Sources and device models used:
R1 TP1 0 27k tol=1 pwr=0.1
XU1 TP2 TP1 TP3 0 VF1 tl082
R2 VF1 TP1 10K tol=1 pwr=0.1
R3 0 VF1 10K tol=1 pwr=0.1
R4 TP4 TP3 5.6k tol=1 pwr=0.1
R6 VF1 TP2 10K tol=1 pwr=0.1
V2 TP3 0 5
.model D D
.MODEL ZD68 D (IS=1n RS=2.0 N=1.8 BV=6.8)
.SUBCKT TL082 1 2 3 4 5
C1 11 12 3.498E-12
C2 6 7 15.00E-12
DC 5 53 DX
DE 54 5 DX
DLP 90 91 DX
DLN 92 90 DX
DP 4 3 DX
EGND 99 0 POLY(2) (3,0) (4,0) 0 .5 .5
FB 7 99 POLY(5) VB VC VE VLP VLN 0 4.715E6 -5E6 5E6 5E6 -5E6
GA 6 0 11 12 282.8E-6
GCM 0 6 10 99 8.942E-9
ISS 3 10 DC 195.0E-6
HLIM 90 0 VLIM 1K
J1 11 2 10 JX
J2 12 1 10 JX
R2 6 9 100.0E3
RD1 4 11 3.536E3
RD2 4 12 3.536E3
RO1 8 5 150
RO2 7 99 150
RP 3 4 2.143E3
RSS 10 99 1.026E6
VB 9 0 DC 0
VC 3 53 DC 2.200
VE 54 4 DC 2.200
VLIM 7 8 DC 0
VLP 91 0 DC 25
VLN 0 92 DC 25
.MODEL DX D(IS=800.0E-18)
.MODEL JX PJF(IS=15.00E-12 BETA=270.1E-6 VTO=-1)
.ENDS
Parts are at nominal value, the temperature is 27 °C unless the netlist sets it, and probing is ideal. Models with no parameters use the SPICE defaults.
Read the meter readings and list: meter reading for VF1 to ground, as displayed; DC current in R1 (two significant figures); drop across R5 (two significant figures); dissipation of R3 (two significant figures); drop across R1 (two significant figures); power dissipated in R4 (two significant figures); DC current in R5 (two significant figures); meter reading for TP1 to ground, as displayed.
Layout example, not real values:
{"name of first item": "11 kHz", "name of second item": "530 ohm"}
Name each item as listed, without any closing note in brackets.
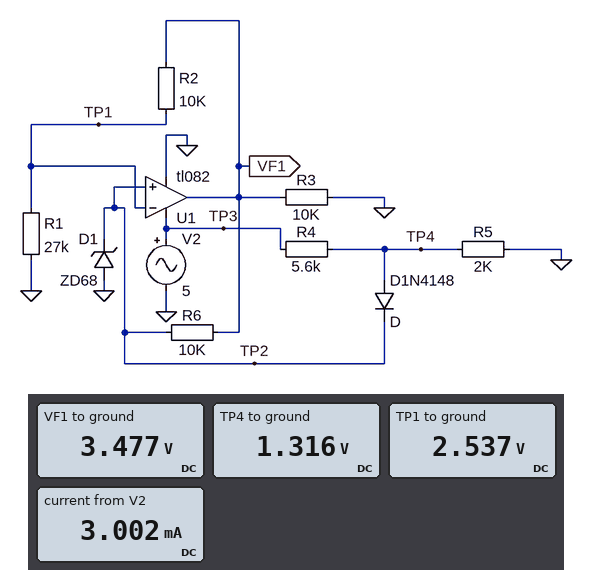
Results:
{"meter reading for VF1 to ground, as displayed": "3.477 V", "DC current in R1": "94 µA", "drop across R5": "1.3 V", "dissipation of R3": "1.2 mW", "drop across R1": "2.5 V", "power dissipated in R4": "2.4 mW", "DC current in R5": "660 µA", "meter reading for TP1 to ground, as displayed": "2.537 V"}
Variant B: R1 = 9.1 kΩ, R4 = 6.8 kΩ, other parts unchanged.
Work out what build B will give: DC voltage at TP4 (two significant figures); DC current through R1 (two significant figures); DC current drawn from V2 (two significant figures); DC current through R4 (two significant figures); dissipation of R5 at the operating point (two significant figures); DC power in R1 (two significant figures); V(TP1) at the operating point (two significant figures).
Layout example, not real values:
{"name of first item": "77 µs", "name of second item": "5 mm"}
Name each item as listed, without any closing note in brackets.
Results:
{"DC voltage at TP4": "1.1 V", "DC current through R1": "180 µA", "DC current drawn from V2": "2.9 mA", "DC current through R4": "570 µA", "dissipation of R5 at the operating point": "650 µW", "DC power in R1": "300 µW", "V(TP1) at the operating point": "1.7 V"}
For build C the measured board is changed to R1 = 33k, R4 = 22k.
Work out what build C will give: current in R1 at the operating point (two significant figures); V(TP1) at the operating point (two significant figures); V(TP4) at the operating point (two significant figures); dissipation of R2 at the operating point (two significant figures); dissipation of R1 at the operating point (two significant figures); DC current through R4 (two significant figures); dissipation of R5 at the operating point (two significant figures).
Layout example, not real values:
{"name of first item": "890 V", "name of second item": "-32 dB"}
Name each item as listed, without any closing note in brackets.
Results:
{"current in R1 at the operating point": "81 µA", "V(TP1) at the operating point": "2.7 V", "V(TP4) at the operating point": "420 mV", "dissipation of R2 at the operating point": "65 µW", "dissipation of R1 at the operating point": "220 µW", "DC current through R4": "210 µA", "dissipation of R5 at the operating point": "87 µW"}
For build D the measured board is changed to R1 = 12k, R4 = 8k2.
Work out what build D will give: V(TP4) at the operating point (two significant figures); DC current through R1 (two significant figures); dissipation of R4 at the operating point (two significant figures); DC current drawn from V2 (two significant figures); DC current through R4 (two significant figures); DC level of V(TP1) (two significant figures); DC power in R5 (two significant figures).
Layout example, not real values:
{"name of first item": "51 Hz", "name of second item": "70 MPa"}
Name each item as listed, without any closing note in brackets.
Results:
{"V(TP4) at the operating point": "980 mV", "DC current through R1": "160 µA", "dissipation of R4 at the operating point": "2.0 mW", "DC current drawn from V2": "2.8 mA", "DC current through R4": "490 µA", "DC level of V(TP1)": "1.9 V", "DC power in R5": "480 µW"}
